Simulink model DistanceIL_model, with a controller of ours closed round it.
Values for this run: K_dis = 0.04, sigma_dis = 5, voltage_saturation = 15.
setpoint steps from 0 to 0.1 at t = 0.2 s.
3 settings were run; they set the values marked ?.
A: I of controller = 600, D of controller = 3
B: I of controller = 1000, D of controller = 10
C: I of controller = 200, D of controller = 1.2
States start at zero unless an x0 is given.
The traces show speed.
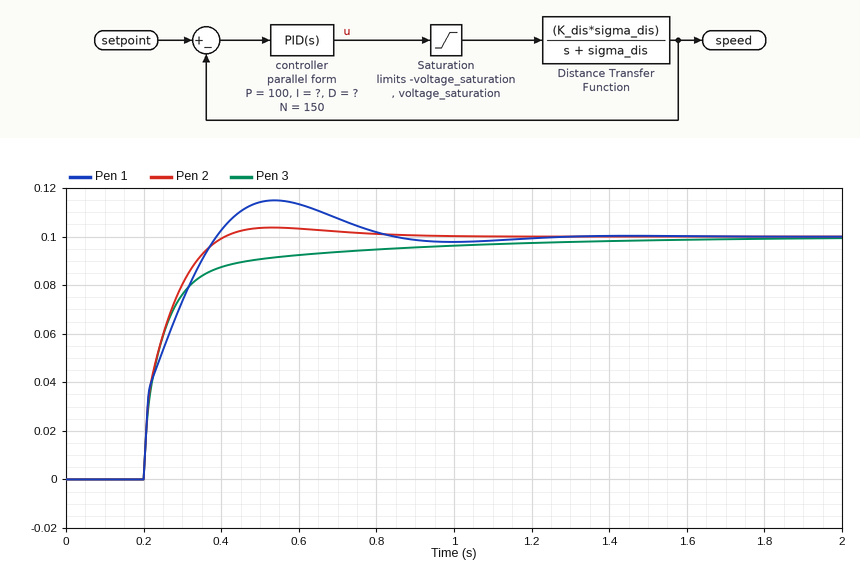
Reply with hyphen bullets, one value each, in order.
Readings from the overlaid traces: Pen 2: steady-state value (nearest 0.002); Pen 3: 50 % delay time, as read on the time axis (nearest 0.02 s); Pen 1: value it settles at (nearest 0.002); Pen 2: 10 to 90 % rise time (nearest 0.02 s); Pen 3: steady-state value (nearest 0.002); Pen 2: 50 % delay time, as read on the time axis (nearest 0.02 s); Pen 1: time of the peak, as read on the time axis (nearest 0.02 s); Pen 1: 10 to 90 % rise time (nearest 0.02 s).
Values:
- 0.100
- 0.24 s
- 0.100
- 0.14 s
- 0.100
- 0.24 s
- 0.54 s
- 0.14 s
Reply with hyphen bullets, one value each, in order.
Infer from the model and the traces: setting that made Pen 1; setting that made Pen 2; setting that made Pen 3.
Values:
- B
- A
- C
